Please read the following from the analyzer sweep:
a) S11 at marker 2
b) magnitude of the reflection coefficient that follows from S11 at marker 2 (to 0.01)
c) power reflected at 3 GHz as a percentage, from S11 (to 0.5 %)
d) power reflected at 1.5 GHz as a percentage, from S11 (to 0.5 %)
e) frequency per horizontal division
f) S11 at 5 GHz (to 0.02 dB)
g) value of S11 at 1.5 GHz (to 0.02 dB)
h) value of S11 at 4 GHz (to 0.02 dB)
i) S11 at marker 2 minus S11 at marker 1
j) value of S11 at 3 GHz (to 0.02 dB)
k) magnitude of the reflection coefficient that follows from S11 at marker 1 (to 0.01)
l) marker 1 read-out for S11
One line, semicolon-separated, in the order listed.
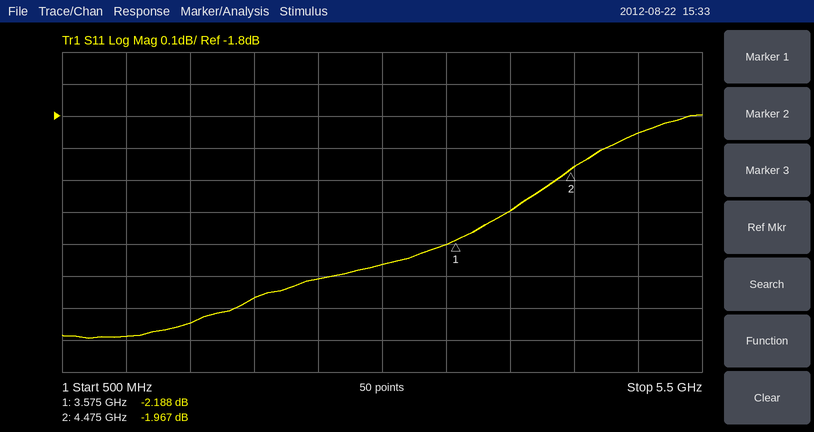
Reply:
-1.967 dB; 0.80; 59.5 %; 57.0 %; 500 MHz; -1.86 dB; -2.44 dB; -2.10 dB; 0.221 dB; -2.26 dB; 0.78; -2.188 dB
